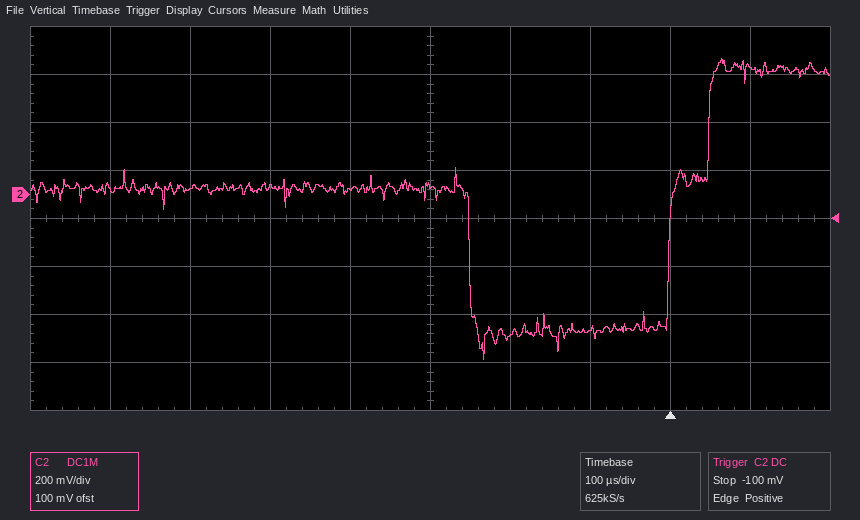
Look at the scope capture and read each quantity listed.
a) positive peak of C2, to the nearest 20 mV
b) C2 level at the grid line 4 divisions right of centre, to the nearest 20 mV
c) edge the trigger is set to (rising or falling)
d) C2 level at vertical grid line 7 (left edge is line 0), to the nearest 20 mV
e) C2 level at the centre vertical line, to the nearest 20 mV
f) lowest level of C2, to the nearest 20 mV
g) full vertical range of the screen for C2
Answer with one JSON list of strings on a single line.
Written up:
["560 mV", "540 mV", "rising", "-560 mV", "40 mV", "-680 mV", "1.6 V"]
